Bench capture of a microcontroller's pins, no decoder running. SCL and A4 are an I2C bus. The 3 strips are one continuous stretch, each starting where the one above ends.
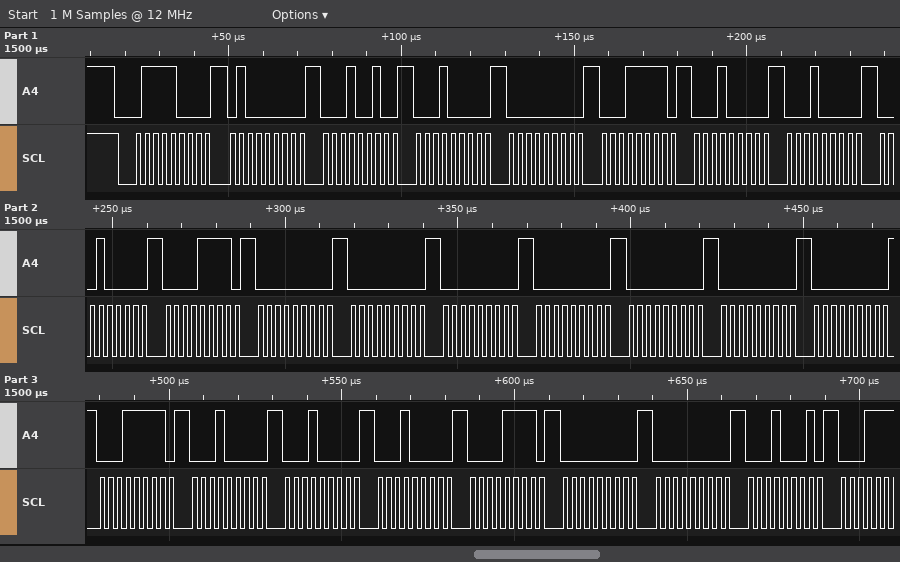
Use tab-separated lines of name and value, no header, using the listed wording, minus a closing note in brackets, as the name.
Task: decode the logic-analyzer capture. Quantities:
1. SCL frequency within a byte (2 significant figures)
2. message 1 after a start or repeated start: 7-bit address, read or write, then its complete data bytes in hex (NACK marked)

SCL frequency within a byte	400 kHz
message 1 after a start or repeated start: 7-bit address, read or write, then its complete data bytes in hex	0x3C write: 40 12 10 00 1F 10 10 10 0F 00 00 00 00 00 00 00 1F 10 10 10 0F 00 00 11
